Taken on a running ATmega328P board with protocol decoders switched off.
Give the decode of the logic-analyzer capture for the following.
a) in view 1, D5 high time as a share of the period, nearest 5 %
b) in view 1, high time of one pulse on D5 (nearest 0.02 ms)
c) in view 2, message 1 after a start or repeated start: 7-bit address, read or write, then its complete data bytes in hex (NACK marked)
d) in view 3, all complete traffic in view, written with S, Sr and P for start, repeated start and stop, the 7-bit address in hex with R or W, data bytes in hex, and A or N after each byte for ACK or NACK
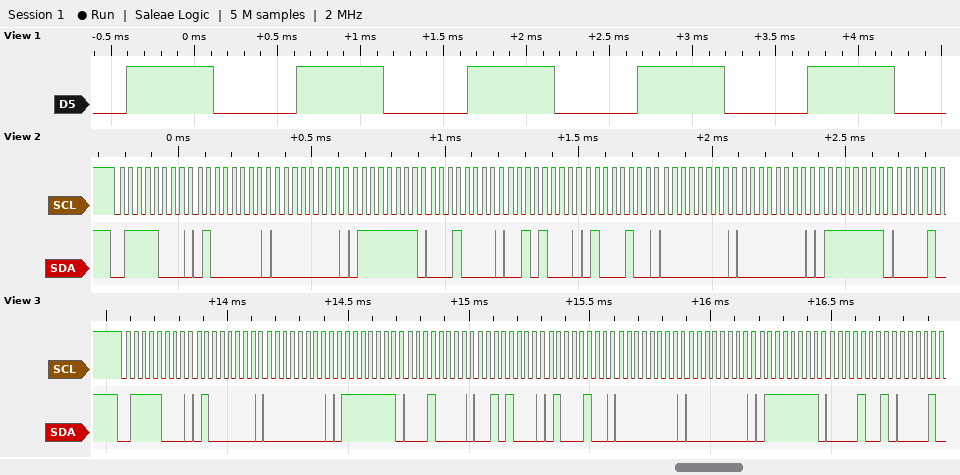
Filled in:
50 %
0.52 ms
0x3C write: 40 00 7F 10 28 44 00 00 7F
S 3CW A 40 A 00 A 7F A 10 A 28 A 44 A 00 A 00 A 7F A 09 A
